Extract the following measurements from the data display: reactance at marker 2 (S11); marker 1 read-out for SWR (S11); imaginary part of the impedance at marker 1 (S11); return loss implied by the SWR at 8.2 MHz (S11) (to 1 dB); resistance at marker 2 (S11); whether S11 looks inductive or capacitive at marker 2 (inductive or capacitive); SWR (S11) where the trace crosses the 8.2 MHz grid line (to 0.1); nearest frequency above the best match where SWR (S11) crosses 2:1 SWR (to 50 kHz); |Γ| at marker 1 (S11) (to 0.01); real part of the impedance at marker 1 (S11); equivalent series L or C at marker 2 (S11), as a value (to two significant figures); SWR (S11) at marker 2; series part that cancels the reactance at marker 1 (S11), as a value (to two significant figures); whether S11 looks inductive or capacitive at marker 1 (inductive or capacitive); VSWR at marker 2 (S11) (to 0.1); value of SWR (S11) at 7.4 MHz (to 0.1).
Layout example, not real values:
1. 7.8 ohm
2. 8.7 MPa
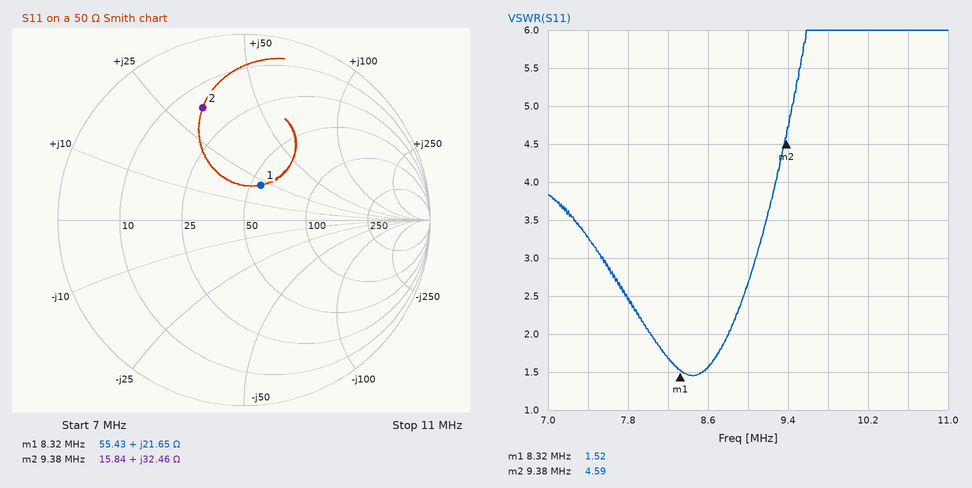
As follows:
1. +32.46 Ω
2. 1.52
3. +21.65 Ω
4. 12 dB
5. 15.84 Ω
6. inductive
7. 1.7
8. 8.80 MHz
9. 0.21
10. 55.43 Ω
11. 550 nH
12. 4.59
13. 880 pF
14. inductive
15. 4.6
16. 3.3
